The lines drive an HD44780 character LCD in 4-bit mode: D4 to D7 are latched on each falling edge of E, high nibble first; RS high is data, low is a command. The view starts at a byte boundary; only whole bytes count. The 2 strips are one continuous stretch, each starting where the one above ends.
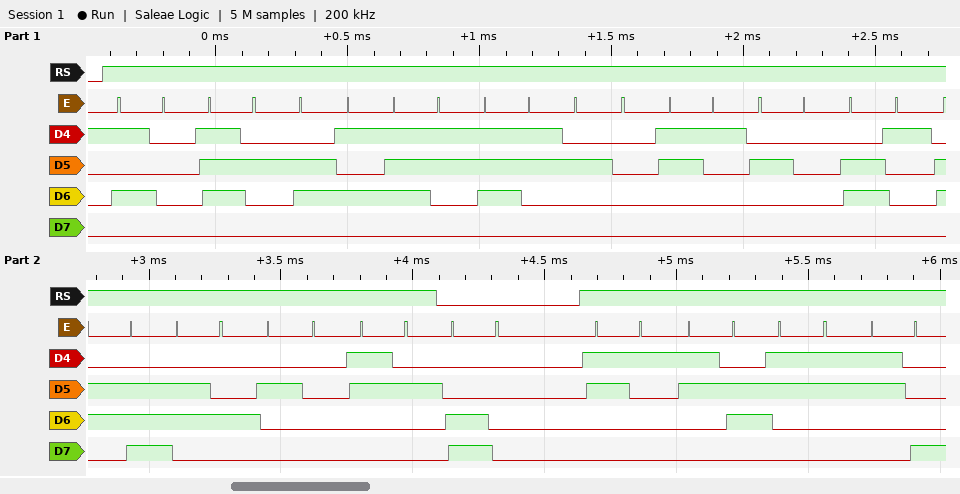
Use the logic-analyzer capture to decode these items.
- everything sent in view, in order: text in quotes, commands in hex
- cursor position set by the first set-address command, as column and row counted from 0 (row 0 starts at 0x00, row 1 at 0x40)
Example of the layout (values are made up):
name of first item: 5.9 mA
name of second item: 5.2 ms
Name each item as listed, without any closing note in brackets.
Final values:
everything sent in view, in order: text in quotes, commands in hex: "Press 1 and 2" 0xC0 "1638"
cursor position set by the first set-address command, as column and row counted from 0: column 0, row 1
